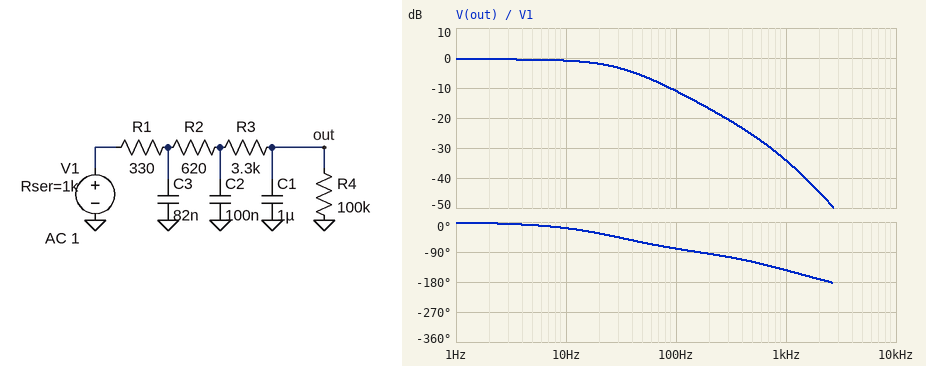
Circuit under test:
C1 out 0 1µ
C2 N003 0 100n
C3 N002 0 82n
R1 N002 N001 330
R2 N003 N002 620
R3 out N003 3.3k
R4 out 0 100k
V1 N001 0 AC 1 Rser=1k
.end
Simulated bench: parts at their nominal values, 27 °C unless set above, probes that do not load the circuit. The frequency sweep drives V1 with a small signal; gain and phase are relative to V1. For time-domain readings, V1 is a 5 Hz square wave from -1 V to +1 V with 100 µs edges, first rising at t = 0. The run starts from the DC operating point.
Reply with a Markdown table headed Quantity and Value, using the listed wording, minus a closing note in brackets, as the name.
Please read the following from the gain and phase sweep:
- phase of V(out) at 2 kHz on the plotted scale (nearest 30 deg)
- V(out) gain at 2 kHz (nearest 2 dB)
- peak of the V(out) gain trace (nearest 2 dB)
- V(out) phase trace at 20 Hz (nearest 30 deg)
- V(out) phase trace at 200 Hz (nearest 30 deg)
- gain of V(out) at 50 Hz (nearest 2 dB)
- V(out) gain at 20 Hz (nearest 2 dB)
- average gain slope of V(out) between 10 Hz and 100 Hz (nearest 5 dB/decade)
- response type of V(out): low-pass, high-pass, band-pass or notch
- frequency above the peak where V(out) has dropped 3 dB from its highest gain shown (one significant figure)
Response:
| Quantity | Value |
|---|---|
| phase of V(out) at 2 kHz on the plotted scale | -180 deg |
| V(out) gain at 2 kHz | -44 dB |
| peak of the V(out) gain trace | 0 dB |
| V(out) phase trace at 20 Hz | -30 deg |
| V(out) phase trace at 200 Hz | -90 deg |
| gain of V(out) at 50 Hz | -6 dB |
| V(out) gain at 20 Hz | -2 dB |
| average gain slope of V(out) between 10 Hz and 100 Hz | -10 dB/decade |
| response type of V(out): low-pass, high-pass, band-pass or notch | low-pass |
| frequency above the peak where V(out) has dropped 3 dB from its highest gain shown | 30 Hz |
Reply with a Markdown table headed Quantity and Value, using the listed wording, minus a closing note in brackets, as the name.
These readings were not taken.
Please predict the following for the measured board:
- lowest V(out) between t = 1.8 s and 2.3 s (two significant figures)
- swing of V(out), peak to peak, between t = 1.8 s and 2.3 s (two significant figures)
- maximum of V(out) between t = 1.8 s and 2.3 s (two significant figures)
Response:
| Quantity | Value |
|---|---|
| lowest V(out) between t = 1.8 s and 2.3 s | -950 mV |
| swing of V(out), peak to peak, between t = 1.8 s and 2.3 s | 1.9 V |
| maximum of V(out) between t = 1.8 s and 2.3 s | 950 mV |
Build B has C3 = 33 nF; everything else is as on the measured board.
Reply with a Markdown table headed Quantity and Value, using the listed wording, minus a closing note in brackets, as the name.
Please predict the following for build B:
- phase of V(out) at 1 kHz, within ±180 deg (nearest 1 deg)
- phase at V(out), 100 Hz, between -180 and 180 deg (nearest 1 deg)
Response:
| Quantity | Value |
|---|---|
| phase of V(out) at 1 kHz, within ±180 deg | -134 deg |
| phase at V(out), 100 Hz, between -180 and 180 deg | -78 deg |
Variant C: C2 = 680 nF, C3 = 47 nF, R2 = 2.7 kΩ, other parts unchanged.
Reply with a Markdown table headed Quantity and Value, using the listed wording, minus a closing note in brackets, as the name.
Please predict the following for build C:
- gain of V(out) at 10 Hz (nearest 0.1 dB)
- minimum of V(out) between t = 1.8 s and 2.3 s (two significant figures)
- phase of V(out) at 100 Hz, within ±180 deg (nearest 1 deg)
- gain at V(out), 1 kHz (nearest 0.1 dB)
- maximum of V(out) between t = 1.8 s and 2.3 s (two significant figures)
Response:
| Quantity | Value |
|---|---|
| gain of V(out) at 10 Hz | -1.7 dB |
| minimum of V(out) between t = 1.8 s and 2.3 s | -930 mV |
| phase of V(out) at 100 Hz, within ±180 deg | -113 deg |
| gain at V(out), 1 kHz | -51.5 dB |
| maximum of V(out) between t = 1.8 s and 2.3 s | 930 mV |
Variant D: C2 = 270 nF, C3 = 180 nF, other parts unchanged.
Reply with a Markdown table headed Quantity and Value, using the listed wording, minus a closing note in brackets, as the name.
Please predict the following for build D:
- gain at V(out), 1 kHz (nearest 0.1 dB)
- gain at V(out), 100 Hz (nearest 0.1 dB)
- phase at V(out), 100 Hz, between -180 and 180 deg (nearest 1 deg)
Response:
| Quantity | Value |
|---|---|
| gain at V(out), 1 kHz | -40.5 dB |
| gain at V(out), 100 Hz | -11.5 dB |
| phase at V(out), 100 Hz, between -180 and 180 deg | -90 deg |
